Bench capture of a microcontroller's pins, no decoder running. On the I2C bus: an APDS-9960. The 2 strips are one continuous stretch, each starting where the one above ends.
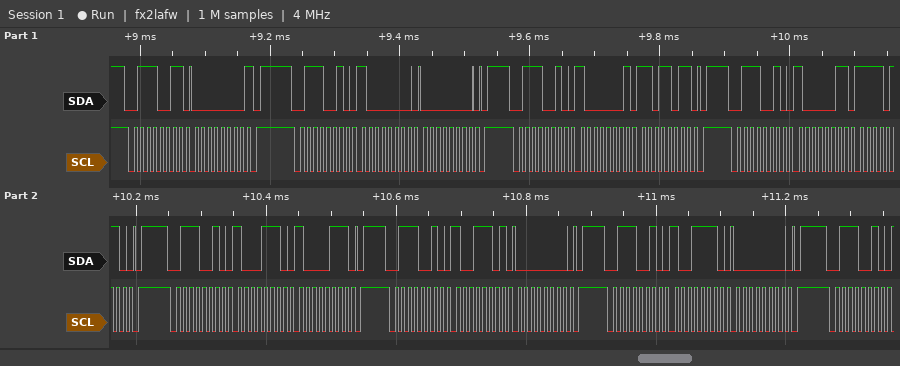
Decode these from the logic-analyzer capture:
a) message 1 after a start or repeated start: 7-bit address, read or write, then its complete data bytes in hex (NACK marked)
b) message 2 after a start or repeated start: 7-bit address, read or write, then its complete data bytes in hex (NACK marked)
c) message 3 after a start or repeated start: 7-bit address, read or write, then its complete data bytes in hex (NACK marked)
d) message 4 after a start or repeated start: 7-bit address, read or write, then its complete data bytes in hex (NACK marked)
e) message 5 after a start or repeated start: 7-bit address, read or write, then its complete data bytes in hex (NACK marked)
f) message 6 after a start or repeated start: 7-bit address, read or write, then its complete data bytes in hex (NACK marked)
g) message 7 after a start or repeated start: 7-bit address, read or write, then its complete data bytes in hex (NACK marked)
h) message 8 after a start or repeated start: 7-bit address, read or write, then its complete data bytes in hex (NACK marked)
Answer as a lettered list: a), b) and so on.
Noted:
a) 0x39 read: 00 NACK
b) 0x39 write: 80 00
c) 0x39 write: 81 DB
d) 0x39 write: 83 F6
e) 0x39 write: 8E 87
f) 0x39 write: 9D 00
g) 0x39 write: 9E 00
h) 0x39 write
